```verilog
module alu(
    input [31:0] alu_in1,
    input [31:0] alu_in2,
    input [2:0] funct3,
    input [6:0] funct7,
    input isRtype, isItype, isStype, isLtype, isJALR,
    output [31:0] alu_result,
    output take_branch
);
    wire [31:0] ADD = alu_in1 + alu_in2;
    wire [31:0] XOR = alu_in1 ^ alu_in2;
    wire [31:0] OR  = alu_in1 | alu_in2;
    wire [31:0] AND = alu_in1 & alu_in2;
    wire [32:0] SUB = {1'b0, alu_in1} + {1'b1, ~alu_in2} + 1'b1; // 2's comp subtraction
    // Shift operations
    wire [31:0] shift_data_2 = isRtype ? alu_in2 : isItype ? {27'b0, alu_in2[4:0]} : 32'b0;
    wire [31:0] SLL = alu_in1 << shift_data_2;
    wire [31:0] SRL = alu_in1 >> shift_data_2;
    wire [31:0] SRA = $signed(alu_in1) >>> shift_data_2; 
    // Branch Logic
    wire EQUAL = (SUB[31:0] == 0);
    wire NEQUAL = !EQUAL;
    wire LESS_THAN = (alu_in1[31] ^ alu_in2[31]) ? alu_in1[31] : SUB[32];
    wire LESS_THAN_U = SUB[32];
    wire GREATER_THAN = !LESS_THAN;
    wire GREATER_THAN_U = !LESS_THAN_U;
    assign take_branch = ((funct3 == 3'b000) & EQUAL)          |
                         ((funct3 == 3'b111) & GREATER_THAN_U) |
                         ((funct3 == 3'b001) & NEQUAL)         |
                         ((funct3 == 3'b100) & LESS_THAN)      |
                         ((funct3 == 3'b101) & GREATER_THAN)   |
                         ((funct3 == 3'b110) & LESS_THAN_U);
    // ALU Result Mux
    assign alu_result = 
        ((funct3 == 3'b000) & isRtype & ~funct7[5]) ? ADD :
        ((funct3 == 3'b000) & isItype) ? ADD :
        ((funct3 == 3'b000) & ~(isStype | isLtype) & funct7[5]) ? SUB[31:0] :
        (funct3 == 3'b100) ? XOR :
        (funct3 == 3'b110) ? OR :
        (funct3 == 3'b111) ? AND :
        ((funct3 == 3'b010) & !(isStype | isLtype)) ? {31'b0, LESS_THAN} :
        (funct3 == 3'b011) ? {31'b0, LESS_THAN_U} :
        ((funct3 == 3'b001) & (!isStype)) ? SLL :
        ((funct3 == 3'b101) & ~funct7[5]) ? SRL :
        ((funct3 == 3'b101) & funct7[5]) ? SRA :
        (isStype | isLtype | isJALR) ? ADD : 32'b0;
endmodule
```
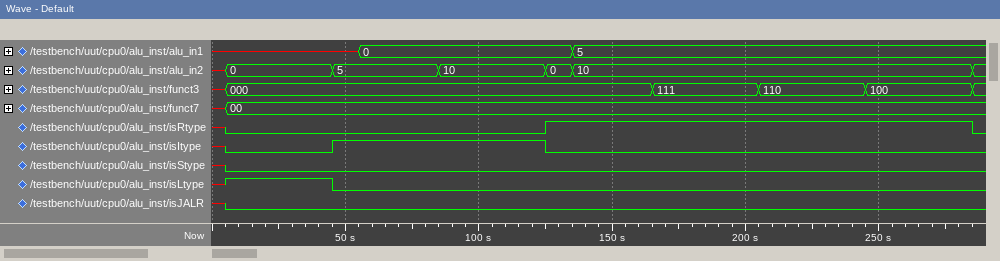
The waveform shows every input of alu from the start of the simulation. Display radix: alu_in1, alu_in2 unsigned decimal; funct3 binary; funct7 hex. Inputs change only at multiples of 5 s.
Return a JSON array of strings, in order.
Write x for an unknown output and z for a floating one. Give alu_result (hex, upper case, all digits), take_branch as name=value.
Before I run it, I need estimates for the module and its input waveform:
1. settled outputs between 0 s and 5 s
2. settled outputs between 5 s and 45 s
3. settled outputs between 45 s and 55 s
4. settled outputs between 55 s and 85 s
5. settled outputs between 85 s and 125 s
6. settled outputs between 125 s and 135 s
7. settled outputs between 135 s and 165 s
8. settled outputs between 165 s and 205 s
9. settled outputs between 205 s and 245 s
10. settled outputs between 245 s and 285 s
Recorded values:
["alu_result=x, take_branch=x", "alu_result=x, take_branch=x", "alu_result=x, take_branch=x", "alu_result=00000005, take_branch=0", "alu_result=0000000A, take_branch=0", "alu_result=00000000, take_branch=1", "alu_result=0000000F, take_branch=0", "alu_result=00000000, take_branch=0", "alu_result=0000000F, take_branch=1", "alu_result=0000000F, take_branch=1"]
